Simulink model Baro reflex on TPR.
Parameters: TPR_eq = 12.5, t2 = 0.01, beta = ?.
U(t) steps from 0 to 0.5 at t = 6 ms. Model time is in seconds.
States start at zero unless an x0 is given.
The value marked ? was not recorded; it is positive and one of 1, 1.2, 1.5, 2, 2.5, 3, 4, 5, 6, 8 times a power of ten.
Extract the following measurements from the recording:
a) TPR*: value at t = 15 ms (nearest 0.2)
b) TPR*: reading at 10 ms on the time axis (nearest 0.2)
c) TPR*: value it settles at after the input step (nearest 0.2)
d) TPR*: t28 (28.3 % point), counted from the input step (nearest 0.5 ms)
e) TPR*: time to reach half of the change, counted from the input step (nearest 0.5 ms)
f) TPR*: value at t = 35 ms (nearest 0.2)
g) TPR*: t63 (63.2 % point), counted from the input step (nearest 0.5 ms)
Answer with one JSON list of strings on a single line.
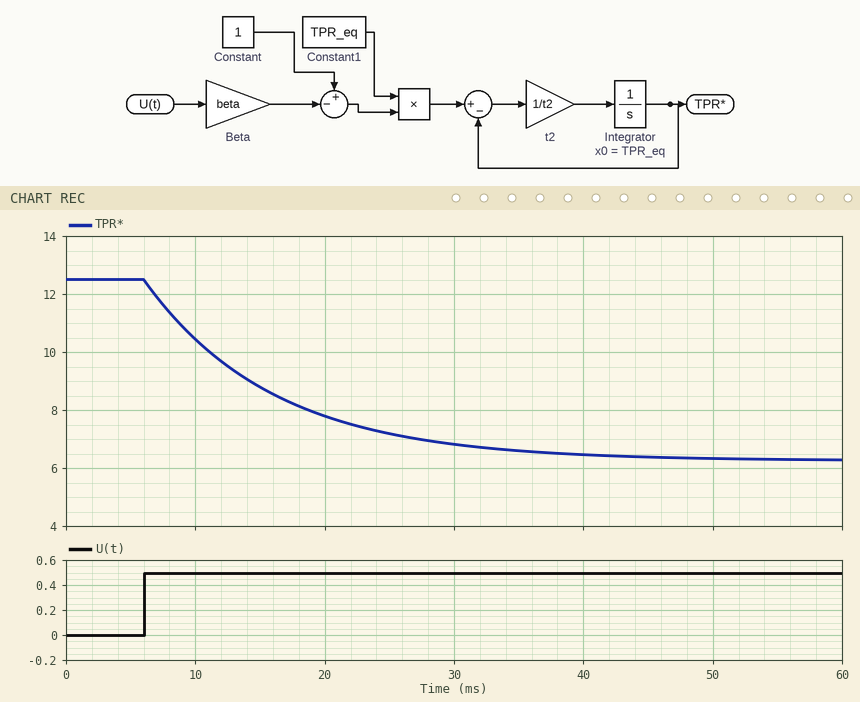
["8.8", "10.4", "6.2", "3.5 ms", "7.0 ms", "6.6", "10.0 ms"]
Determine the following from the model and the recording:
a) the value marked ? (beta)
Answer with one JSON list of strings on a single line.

["1"]
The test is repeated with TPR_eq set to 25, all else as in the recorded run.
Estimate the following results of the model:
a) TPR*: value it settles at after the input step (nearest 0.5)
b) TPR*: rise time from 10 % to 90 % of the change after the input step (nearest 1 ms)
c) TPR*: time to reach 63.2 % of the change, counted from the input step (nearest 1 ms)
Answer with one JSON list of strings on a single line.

["12.5", "22 ms", "10 ms"]
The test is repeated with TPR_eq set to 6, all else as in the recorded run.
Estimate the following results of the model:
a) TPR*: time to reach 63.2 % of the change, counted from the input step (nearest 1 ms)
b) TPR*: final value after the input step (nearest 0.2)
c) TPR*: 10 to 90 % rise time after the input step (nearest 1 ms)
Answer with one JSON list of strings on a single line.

["10 ms", "3.0", "22 ms"]
